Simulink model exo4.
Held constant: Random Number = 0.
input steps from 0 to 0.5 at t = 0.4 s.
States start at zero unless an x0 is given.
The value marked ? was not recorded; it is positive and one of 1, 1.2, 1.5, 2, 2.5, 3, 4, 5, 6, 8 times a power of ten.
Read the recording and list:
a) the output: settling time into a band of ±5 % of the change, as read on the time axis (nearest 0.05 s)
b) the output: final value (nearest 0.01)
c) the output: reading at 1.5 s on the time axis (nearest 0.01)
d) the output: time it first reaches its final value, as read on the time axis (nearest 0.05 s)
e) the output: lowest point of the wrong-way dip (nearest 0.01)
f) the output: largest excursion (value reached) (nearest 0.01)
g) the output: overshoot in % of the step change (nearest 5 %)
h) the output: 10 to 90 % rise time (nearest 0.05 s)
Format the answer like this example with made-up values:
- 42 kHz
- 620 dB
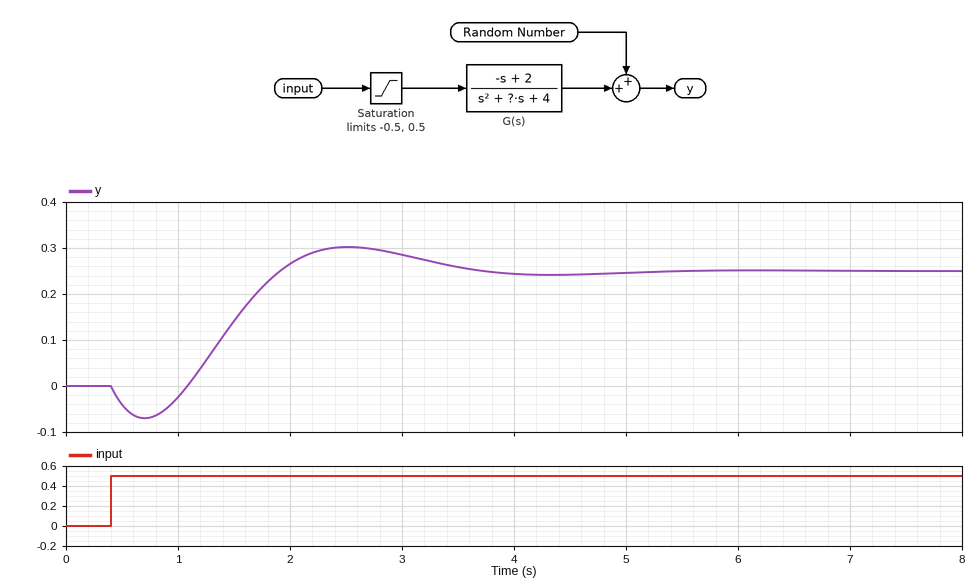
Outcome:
- 3.40 s
- 0.25
- 0.14
- 1.90 s
- -0.07
- 0.30
- 20 %
- 0.65 s
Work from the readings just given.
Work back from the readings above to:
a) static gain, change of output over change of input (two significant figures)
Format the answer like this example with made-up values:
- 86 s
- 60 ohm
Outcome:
- 0.50
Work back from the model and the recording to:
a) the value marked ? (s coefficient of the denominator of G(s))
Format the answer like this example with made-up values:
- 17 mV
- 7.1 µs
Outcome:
- 2
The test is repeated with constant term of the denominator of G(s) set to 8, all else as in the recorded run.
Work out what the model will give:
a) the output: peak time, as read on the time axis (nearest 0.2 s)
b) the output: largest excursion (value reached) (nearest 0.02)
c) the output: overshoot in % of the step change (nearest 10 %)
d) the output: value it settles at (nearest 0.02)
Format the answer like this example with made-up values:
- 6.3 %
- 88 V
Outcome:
- 1.8 s
- 0.18
- 50 %
- 0.12
